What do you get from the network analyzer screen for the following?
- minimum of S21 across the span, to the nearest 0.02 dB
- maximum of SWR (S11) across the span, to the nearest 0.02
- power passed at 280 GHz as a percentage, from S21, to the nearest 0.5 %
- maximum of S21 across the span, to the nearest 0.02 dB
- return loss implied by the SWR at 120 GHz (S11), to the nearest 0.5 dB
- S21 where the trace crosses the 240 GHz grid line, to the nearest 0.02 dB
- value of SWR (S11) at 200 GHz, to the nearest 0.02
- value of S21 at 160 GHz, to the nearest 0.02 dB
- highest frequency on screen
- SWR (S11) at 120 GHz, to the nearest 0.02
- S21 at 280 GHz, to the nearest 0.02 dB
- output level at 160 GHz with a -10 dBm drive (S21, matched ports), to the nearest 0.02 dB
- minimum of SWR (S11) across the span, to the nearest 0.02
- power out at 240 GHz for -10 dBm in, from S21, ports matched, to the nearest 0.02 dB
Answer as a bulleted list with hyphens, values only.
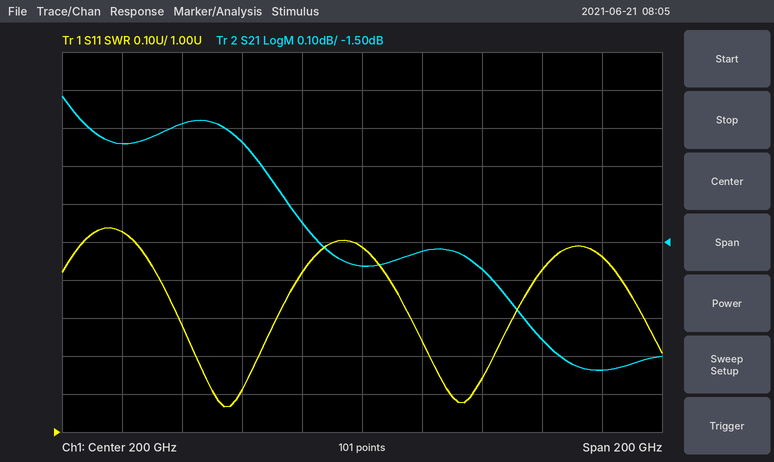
- -1.84 dB
- 1.54
- 65.5 %
- -1.12 dB
- 13.5 dB
- -1.58 dB
- 1.48
- -1.24 dB
- 300 GHz
- 1.52
- -1.84 dB
- -11.24 dBm
- 1.06
- -11.58 dBm
